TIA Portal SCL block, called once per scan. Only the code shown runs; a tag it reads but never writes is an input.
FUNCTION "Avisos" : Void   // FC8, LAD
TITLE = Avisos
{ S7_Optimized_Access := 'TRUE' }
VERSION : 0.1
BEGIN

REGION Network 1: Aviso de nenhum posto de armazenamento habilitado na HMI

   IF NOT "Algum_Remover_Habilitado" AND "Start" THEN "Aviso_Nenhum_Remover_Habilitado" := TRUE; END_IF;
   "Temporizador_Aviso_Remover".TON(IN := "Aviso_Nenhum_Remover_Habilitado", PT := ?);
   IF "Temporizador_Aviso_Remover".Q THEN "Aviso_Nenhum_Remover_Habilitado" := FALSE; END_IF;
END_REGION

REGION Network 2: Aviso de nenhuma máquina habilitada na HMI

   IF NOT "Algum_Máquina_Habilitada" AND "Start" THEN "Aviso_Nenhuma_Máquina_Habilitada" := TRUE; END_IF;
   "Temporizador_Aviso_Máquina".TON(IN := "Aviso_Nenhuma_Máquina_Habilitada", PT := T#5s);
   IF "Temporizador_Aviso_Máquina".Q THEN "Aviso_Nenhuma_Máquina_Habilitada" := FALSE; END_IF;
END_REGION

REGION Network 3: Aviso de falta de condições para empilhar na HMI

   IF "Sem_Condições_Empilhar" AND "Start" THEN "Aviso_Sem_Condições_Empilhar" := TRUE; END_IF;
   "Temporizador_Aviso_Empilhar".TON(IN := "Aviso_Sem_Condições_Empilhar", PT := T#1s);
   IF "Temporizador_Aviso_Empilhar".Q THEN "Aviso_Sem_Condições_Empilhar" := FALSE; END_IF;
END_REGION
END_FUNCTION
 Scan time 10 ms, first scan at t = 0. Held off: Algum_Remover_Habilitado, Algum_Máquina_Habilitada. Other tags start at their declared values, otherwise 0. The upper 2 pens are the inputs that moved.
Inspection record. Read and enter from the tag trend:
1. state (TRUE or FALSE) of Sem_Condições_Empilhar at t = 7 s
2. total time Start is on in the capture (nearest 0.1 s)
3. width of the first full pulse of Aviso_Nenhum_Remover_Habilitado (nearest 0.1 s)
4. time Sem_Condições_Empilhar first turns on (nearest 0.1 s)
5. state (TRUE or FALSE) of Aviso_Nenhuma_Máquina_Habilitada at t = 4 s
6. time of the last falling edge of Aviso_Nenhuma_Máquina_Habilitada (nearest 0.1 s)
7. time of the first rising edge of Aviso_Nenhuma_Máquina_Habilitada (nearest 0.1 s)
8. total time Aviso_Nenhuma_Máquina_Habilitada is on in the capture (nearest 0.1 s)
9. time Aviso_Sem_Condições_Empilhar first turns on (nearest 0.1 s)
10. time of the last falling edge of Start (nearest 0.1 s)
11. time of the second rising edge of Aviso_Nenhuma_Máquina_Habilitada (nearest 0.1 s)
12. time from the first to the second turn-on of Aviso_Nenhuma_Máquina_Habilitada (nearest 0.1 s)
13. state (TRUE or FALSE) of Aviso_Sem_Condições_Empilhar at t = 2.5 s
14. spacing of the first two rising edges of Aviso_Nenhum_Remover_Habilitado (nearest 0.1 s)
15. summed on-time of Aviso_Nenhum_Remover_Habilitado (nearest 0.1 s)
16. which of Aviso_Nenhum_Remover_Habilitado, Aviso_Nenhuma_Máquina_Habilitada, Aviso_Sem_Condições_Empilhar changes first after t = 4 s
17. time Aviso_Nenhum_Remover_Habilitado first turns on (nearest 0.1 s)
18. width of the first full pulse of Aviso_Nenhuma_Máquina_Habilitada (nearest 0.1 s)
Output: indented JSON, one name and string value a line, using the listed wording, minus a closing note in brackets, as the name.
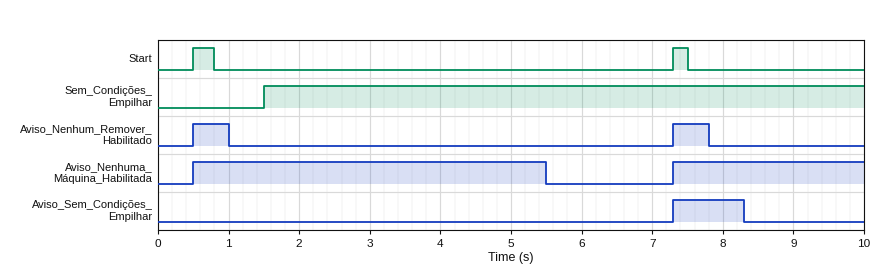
{
  "state (TRUE or FALSE) of Sem_Condições_Empilhar at t = 7 s": "TRUE",
  "total time Start is on in the capture": "0.5 s",
  "width of the first full pulse of Aviso_Nenhum_Remover_Habilitado": "0.5 s",
  "time Sem_Condições_Empilhar first turns on": "1.5 s",
  "state (TRUE or FALSE) of Aviso_Nenhuma_Máquina_Habilitada at t = 4 s": "TRUE",
  "time of the last falling edge of Aviso_Nenhuma_Máquina_Habilitada": "5.5 s",
  "time of the first rising edge of Aviso_Nenhuma_Máquina_Habilitada": "0.5 s",
  "total time Aviso_Nenhuma_Máquina_Habilitada is on in the capture": "7.7 s",
  "time Aviso_Sem_Condições_Empilhar first turns on": "7.3 s",
  "time of the last falling edge of Start": "7.5 s",
  "time of the second rising edge of Aviso_Nenhuma_Máquina_Habilitada": "7.3 s",
  "time from the first to the second turn-on of Aviso_Nenhuma_Máquina_Habilitada": "6.8 s",
  "state (TRUE or FALSE) of Aviso_Sem_Condições_Empilhar at t = 2.5 s": "FALSE",
  "spacing of the first two rising edges of Aviso_Nenhum_Remover_Habilitado": "6.8 s",
  "summed on-time of Aviso_Nenhum_Remover_Habilitado": "1.0 s",
  "which of Aviso_Nenhum_Remover_Habilitado, Aviso_Nenhuma_Máquina_Habilitada, Aviso_Sem_Condições_Empilhar changes first after t = 4 s": "Aviso_Nenhuma_Máquina_Habilitada",
  "time Aviso_Nenhum_Remover_Habilitado first turns on": "0.5 s",
  "width of the first full pulse of Aviso_Nenhuma_Máquina_Habilitada": "5.0 s"
}
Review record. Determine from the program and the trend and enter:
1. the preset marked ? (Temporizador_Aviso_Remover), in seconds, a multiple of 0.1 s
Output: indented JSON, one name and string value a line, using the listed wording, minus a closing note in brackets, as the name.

{
  "the preset marked ? (Temporizador_Aviso_Remover), in seconds, a multiple of 0.1 s": "0.5 s"
}
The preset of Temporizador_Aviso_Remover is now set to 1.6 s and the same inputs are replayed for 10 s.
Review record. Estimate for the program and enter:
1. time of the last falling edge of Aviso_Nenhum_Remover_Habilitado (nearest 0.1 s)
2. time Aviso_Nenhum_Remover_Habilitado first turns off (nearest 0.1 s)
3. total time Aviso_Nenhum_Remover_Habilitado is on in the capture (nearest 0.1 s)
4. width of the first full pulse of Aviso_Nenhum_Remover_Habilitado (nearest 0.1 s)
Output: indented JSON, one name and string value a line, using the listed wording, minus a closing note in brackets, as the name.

{
  "time of the last falling edge of Aviso_Nenhum_Remover_Habilitado": "8.9 s",
  "time Aviso_Nenhum_Remover_Habilitado first turns off": "2.1 s",
  "total time Aviso_Nenhum_Remover_Habilitado is on in the capture": "3.2 s",
  "width of the first full pulse of Aviso_Nenhum_Remover_Habilitado": "1.6 s"
}
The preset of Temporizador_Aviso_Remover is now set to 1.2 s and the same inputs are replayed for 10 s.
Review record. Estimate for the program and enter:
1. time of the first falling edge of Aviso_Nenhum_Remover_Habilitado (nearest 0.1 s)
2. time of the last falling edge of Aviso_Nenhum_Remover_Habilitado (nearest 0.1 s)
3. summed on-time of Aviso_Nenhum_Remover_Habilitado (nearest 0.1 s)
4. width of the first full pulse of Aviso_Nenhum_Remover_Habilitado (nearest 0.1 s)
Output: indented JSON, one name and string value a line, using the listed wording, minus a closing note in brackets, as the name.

{
  "time of the first falling edge of Aviso_Nenhum_Remover_Habilitado": "1.7 s",
  "time of the last falling edge of Aviso_Nenhum_Remover_Habilitado": "8.5 s",
  "summed on-time of Aviso_Nenhum_Remover_Habilitado": "2.4 s",
  "width of the first full pulse of Aviso_Nenhum_Remover_Habilitado": "1.2 s"
}
